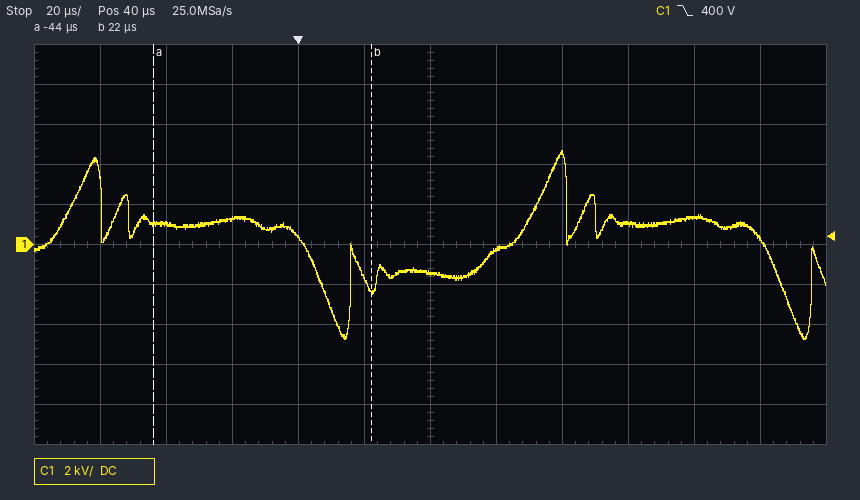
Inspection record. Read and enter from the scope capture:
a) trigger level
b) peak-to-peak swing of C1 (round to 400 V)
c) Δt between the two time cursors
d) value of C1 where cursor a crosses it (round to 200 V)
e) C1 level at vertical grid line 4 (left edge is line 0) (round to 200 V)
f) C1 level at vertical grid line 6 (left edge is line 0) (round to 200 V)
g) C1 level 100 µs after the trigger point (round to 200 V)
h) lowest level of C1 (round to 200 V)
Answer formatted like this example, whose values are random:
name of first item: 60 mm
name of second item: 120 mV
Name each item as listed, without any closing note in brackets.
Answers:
trigger level: 400 V
peak-to-peak swing of C1: 9.6 kV
Δt between the two time cursors: 66 µs
value of C1 where cursor a crosses it: 1.0 kV
C1 level at vertical grid line 4 (left edge is line 0): 400 V
C1 level at vertical grid line 6 (left edge is line 0): -1.4 kV
C1 level 100 µs after the trigger point: 1.0 kV
lowest level of C1: -4.8 kV
